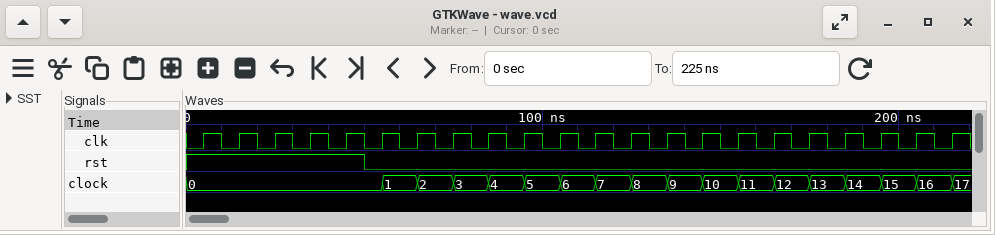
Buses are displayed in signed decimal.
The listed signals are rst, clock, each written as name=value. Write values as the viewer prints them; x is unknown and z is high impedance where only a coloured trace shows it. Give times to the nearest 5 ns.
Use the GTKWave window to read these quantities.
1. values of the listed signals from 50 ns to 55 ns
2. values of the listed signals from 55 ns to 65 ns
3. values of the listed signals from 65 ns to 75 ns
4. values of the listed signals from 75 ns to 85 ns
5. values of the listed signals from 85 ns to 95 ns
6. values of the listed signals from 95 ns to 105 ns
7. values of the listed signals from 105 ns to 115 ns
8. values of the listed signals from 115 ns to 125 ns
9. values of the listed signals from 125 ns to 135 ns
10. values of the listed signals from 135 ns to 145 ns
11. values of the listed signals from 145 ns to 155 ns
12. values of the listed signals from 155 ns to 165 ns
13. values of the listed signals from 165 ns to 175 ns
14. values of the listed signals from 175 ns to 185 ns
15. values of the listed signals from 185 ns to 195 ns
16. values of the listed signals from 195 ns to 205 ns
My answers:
rst=0, clock=0
rst=0, clock=1
rst=0, clock=2
rst=0, clock=3
rst=0, clock=4
rst=0, clock=5
rst=0, clock=6
rst=0, clock=7
rst=0, clock=8
rst=0, clock=9
rst=0, clock=10
rst=0, clock=11
rst=0, clock=12
rst=0, clock=13
rst=0, clock=14
rst=0, clock=15
